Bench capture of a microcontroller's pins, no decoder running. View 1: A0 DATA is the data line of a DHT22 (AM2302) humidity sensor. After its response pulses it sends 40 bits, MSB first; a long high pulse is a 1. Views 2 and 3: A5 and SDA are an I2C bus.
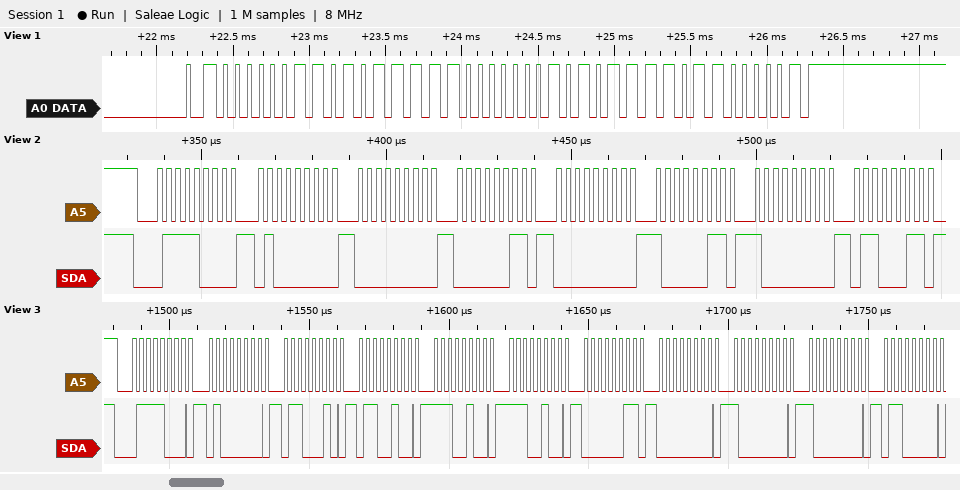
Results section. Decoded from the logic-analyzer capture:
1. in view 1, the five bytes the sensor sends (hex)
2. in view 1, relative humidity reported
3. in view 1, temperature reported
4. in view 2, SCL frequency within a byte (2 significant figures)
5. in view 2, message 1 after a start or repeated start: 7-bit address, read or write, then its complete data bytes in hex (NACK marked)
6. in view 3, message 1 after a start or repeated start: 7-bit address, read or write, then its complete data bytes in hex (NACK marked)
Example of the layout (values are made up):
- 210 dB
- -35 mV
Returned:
- 03 5F 01 5E C1
- 86.3 %
- 35.0 °C
- 400 kHz
- 0x3C write: 40 00 03 00 83 80 63
- 0x3C write: 40 62 64 E4 E4 03 00 80 80 60
